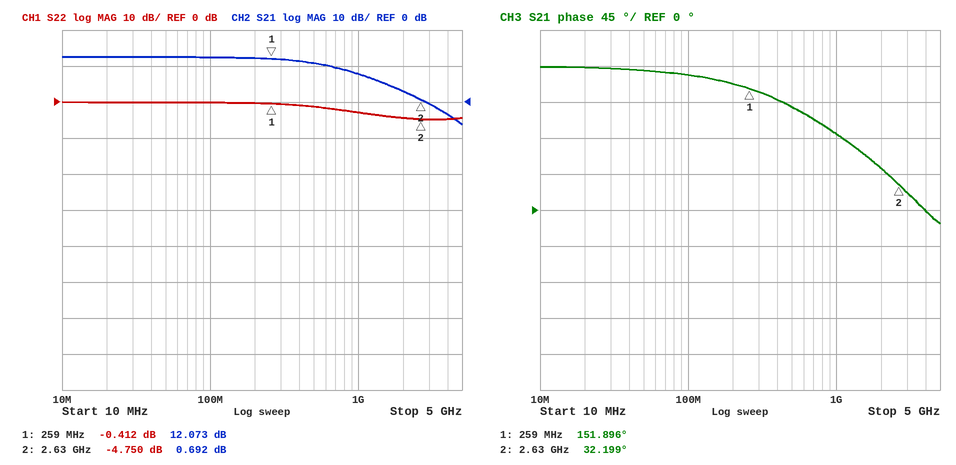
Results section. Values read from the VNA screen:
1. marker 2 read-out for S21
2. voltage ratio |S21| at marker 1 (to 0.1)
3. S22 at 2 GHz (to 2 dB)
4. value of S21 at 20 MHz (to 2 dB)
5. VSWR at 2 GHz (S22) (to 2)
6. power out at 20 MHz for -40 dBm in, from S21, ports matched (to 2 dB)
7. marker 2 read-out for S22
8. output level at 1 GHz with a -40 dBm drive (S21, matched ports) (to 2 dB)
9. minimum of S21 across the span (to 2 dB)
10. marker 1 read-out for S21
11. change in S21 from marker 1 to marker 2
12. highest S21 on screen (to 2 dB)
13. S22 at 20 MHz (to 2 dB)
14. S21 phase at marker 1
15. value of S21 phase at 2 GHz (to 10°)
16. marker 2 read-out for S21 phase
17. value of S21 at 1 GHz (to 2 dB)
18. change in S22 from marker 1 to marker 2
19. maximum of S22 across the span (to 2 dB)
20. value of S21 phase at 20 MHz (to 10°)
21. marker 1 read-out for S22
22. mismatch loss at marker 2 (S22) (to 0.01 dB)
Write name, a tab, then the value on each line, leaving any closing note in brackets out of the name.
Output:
marker 2 read-out for S21	0.692 dB
voltage ratio |S21| at marker 1	4.0
S22 at 2 GHz	-4 dB
value of S21 at 20 MHz	12 dB
VSWR at 2 GHz (S22)	4
power out at 20 MHz for -40 dBm in, from S21, ports matched	-28 dBm
marker 2 read-out for S22	-4.750 dB
output level at 1 GHz with a -40 dBm drive (S21, matched ports)	-32 dBm
minimum of S21 across the span	-6 dB
marker 1 read-out for S21	12.073 dB
change in S21 from marker 1 to marker 2	-11.381 dB
highest S21 on screen	12 dB
S22 at 20 MHz	0 dB
S21 phase at marker 1	151.896°
value of S21 phase at 2 GHz	50°
marker 2 read-out for S21 phase	32.199°
value of S21 at 1 GHz	8 dB
change in S22 from marker 1 to marker 2	-4.338 dB
maximum of S22 across the span	0 dB
value of S21 phase at 20 MHz	180°
marker 1 read-out for S22	-0.412 dB
mismatch loss at marker 2 (S22)	1.77 dB
